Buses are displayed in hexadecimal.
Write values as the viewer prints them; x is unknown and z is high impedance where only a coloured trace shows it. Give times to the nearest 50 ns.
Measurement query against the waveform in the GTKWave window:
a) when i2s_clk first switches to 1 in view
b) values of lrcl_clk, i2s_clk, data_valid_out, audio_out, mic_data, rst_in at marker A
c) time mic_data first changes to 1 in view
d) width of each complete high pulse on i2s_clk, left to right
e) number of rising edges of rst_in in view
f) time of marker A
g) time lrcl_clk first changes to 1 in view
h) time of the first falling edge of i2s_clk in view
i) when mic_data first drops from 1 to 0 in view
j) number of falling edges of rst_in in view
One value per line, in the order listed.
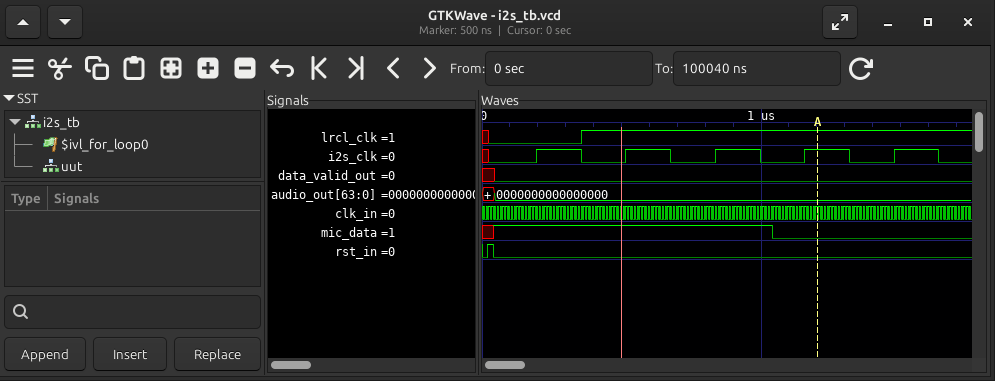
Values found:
200 ns
lrcl_clk=1, i2s_clk=1, data_valid_out=0, audio_out=0000000000000000, mic_data=0, rst_in=0
50 ns
150 ns, 150 ns, 150 ns, 150 ns, 150 ns
1
1200 ns
350 ns
350 ns
1050 ns
1
